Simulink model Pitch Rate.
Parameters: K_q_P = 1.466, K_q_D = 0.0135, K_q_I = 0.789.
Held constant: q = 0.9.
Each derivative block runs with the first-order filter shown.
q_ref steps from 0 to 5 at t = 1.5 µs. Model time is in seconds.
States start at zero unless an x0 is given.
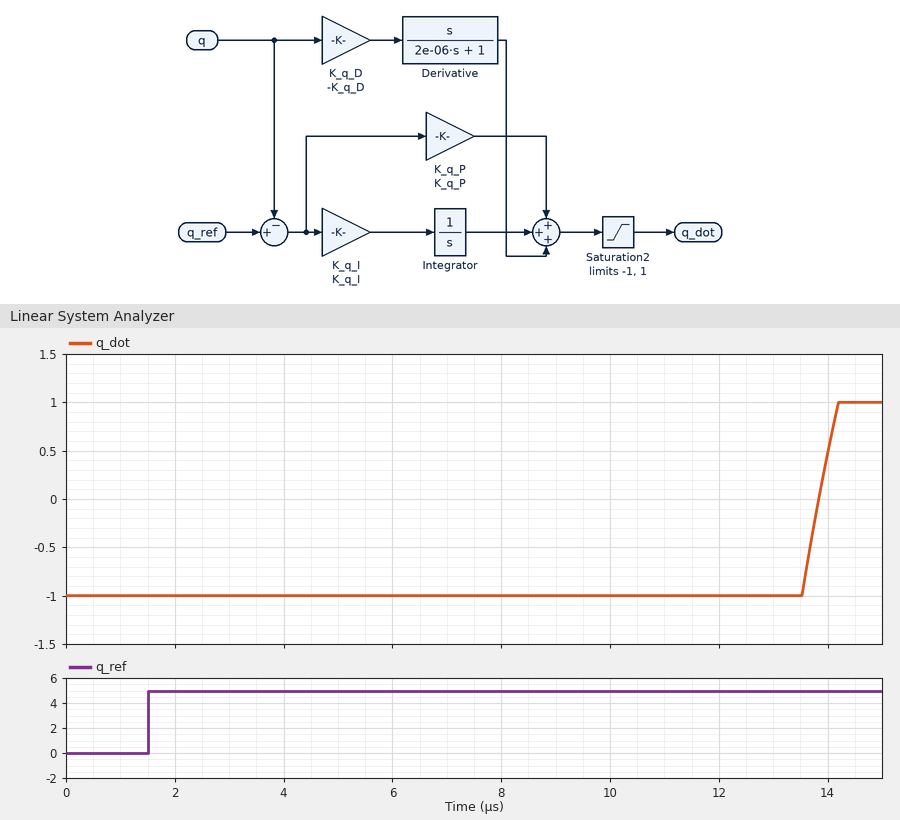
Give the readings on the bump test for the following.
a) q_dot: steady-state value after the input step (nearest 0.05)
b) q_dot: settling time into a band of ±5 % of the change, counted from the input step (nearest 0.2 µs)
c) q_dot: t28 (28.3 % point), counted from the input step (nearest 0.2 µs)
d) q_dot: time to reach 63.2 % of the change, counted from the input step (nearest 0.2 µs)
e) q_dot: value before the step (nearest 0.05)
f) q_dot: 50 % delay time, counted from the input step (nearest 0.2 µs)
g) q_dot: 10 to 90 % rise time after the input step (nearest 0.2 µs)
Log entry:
1.00
12.6 µs
12.2 µs
12.4 µs
-1.00
12.4 µs
0.6 µs
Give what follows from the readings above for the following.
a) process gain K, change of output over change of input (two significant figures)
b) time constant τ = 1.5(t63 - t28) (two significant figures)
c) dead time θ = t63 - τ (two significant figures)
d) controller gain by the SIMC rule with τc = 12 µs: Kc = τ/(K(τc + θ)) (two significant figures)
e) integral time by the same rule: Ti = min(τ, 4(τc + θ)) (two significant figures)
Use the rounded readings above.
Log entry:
0.40
0.30 µs
12 µs
0.031
0.30 µs
